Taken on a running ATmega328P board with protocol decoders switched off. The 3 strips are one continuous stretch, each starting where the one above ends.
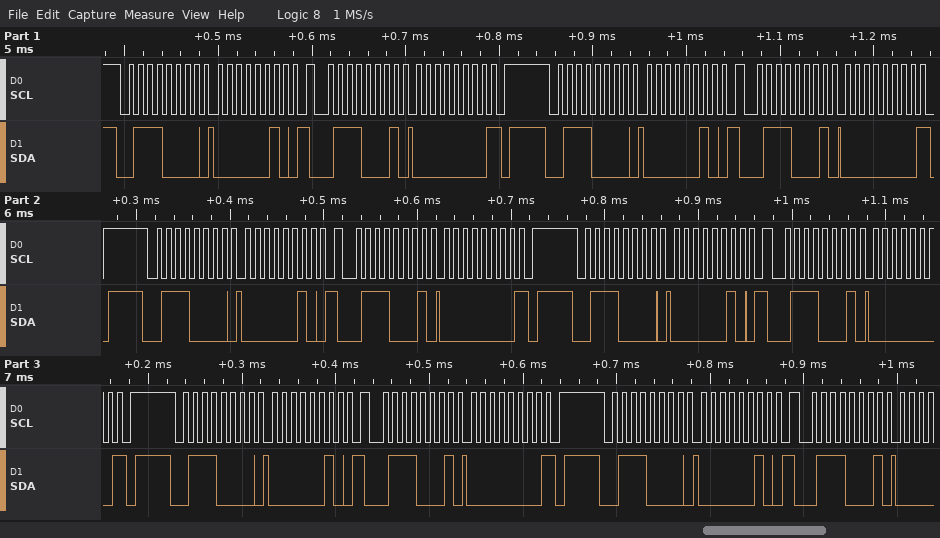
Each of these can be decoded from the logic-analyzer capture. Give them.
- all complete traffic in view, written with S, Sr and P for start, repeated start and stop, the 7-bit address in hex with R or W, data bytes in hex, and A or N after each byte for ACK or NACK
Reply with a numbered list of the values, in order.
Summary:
1. S 38W A 02 A Sr 38R A 00 N P S 38W A 02 A Sr 38R A 00 N P S 38W A 02 A Sr 38R A 00 N P S 38W A 02 A Sr 38R A 00 N P S 38W A 02 A Sr 38R A 00 N P S 38W A 02 A Sr 38R A
